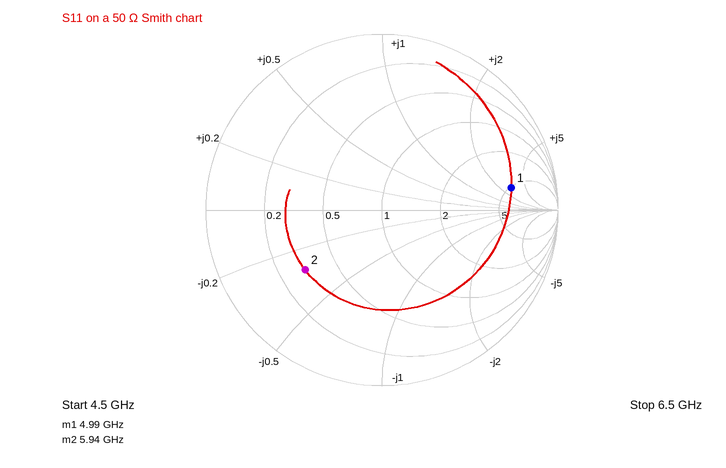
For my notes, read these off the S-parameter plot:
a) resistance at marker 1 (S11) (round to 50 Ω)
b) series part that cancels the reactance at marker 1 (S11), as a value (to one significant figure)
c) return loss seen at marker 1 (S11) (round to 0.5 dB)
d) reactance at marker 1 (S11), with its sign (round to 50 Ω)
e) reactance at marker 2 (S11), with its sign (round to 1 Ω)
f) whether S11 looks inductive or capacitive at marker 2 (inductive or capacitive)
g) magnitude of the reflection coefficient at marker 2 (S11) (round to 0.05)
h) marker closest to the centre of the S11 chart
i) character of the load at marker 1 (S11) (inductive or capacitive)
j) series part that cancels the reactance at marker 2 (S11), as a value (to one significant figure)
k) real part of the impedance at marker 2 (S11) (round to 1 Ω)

250 Ω
200 fF
2.5 dB
+150 Ω
-16 Ω
capacitive
0.55
marker 2
inductive
400 pH
16 Ω
